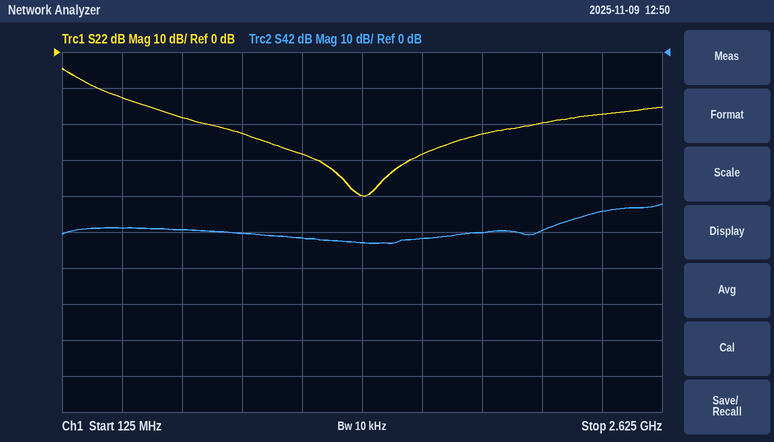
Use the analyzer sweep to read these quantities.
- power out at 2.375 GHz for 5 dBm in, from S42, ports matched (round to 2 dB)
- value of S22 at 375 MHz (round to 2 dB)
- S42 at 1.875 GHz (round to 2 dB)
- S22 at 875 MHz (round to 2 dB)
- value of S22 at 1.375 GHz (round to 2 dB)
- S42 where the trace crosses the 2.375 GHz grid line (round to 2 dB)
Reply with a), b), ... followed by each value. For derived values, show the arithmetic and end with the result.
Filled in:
a) 5 dBm + (-44 dB) = -40 dBm
b) -12 dB
c) -50 dB
d) -22 dB
e) -40 dB
f) -44 dB
